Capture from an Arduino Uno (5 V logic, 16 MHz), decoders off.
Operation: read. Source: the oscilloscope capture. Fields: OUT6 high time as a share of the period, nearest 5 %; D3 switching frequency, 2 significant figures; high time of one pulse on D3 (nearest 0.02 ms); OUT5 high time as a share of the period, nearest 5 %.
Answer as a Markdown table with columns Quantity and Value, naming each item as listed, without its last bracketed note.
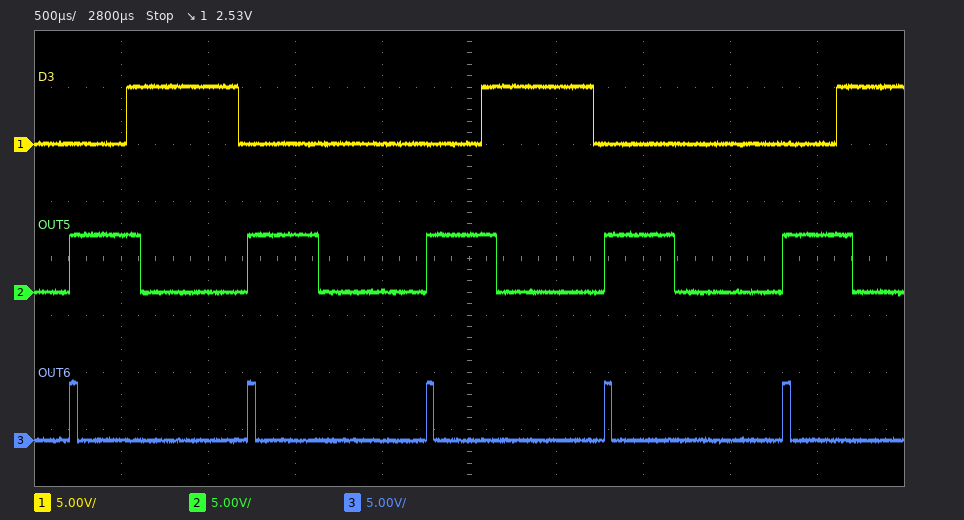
| Quantity | Value |
|---|---|
| OUT6 high time as a share of the period, nearest 5 % | 5 % |
| D3 switching frequency, 2 significant figures | 490 Hz |
| high time of one pulse on D3 | 0.64 ms |
| OUT5 high time as a share of the period, nearest 5 % | 40 % |
